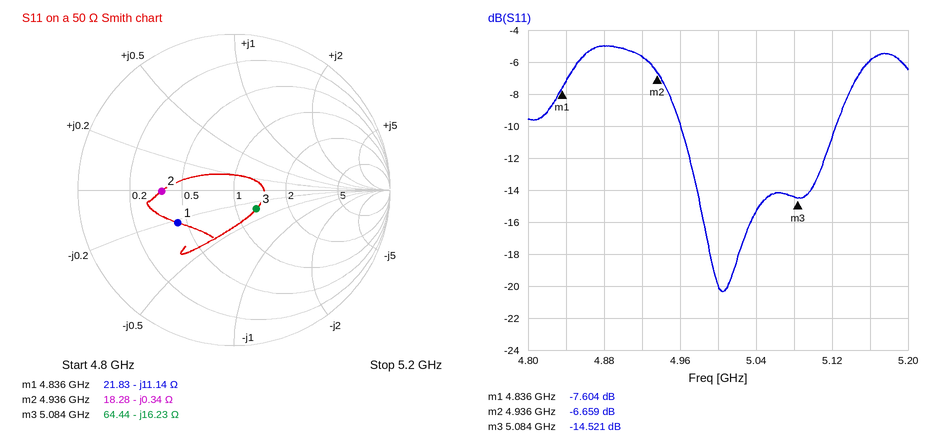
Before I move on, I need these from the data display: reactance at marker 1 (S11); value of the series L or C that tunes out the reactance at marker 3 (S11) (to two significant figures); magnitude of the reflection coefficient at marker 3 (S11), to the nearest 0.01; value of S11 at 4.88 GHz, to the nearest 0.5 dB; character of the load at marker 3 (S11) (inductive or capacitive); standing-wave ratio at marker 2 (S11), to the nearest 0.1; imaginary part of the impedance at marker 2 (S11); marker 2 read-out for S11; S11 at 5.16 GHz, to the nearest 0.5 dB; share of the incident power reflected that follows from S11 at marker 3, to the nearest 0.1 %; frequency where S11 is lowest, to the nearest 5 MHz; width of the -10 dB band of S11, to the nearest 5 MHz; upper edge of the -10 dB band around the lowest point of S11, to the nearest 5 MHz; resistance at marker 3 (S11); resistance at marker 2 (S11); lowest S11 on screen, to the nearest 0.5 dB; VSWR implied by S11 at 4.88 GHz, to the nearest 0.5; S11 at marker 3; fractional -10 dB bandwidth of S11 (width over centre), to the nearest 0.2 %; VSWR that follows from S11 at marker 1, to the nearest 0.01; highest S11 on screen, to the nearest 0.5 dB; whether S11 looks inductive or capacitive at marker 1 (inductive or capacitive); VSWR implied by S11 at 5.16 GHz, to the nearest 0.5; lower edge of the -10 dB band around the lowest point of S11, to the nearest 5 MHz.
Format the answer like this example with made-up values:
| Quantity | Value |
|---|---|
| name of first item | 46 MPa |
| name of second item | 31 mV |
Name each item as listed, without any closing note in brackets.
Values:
| Quantity | Value |
|---|---|
| reactance at marker 1 | -11.14 Ω |
| value of the series L or C that tunes out the reactance at marker 3 (S11) | 510 pH |
| magnitude of the reflection coefficient at marker 3 (S11), to the nearest 0.01 | 0.19 |
| value of S11 at 4.88 GHz, to the nearest 0.5 dB | -5.0 dB |
| character of the load at marker 3 (S11) | capacitive |
| standing-wave ratio at marker 2 (S11), to the nearest 0.1 | 2.7 |
| imaginary part of the impedance at marker 2 | -0.34 Ω |
| marker 2 read-out for S11 | -6.659 dB |
| S11 at 5.16 GHz, to the nearest 0.5 dB | -6.0 dB |
| share of the incident power reflected that follows from S11 at marker 3, to the nearest 0.1 % | 3.5 % |
| frequency where S11 is lowest, to the nearest 5 MHz | 5.005 GHz |
| width of the -10 dB band of S11, to the nearest 5 MHz | 165 MHz |
| upper edge of the -10 dB band around the lowest point of S11, to the nearest 5 MHz | 5.125 GHz |
| resistance at marker 3 | 64.44 Ω |
| resistance at marker 2 | 18.28 Ω |
| lowest S11 on screen, to the nearest 0.5 dB | -20.5 dB |
| VSWR implied by S11 at 4.88 GHz, to the nearest 0.5 | 3.5 |
| S11 at marker 3 | -14.521 dB |
| fractional -10 dB bandwidth of S11 (width over centre), to the nearest 0.2 % | 3.2 % |
| VSWR that follows from S11 at marker 1, to the nearest 0.01 | 2.43 |
| highest S11 on screen, to the nearest 0.5 dB | -5.0 dB |
| whether S11 looks inductive or capacitive at marker 1 | capacitive |
| VSWR implied by S11 at 5.16 GHz, to the nearest 0.5 | 3.0 |
| lower edge of the -10 dB band around the lowest point of S11, to the nearest 5 MHz | 4.960 GHz |
